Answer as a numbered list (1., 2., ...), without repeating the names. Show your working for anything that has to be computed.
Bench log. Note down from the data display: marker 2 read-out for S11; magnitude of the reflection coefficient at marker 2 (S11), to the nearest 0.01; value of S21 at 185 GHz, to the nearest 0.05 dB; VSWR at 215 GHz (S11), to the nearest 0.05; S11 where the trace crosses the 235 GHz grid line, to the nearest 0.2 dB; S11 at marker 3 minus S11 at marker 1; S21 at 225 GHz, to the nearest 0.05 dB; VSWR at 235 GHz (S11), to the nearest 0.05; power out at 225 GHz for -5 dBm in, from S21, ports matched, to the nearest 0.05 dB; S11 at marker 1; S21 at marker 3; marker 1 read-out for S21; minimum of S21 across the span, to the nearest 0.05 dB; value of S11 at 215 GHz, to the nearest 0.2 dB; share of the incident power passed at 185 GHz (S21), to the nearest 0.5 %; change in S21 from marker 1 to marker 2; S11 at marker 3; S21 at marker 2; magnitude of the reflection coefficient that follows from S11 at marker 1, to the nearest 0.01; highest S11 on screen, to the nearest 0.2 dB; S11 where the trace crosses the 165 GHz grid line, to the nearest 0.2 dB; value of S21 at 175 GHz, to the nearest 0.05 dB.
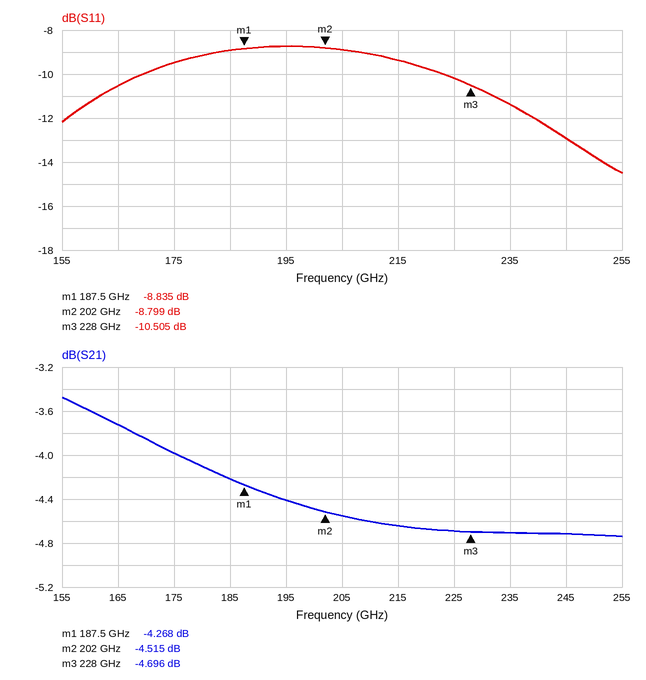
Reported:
1. -8.799 dB
2. 10^(-8.799/20) ≈ 0.36
3. -4.20 dB
4. |Γ| = 10^(-9.4/20) = 0.3388; VSWR = (1 + 0.3388)/(1 − 0.3388) ≈ 2.03, so 2.05 to the nearest 0.05
5. -11.4 dB
6. -10.505 − (-8.835) = -1.670 dB
7. -4.70 dB
8. |Γ| = 10^(-11.4/20) = 0.2692; VSWR = (1 + 0.2692)/(1 − 0.2692) ≈ 1.74, so 1.75 to the nearest 0.05
9. -5 dBm + (-4.70 dB) = -9.70 dBm
10. -8.835 dB
11. -4.696 dB
12. -4.268 dB
13. -4.75 dB
14. -9.4 dB
15. 10^(-4.2/10) ≈ 38.0 %
16. -4.515 − (-4.268) = -0.247 dB
17. -10.505 dB
18. -4.515 dB
19. 10^(-8.835/20) ≈ 0.36
20. -8.8 dB
21. -10.6 dB
22. -4.00 dB
